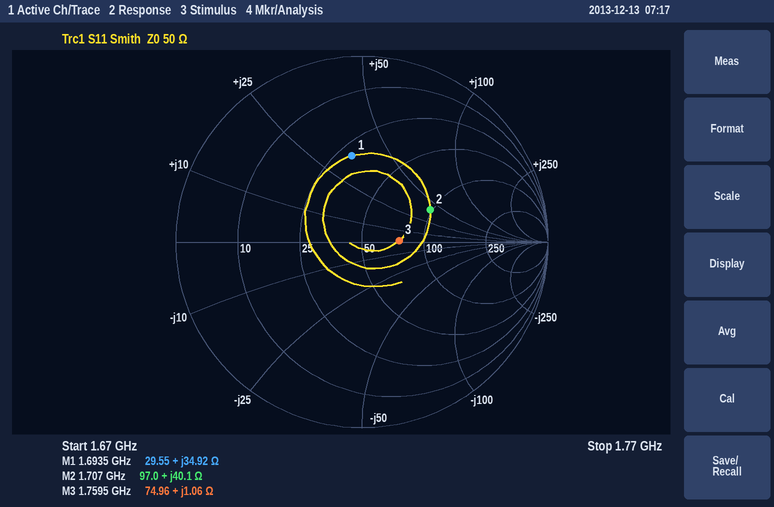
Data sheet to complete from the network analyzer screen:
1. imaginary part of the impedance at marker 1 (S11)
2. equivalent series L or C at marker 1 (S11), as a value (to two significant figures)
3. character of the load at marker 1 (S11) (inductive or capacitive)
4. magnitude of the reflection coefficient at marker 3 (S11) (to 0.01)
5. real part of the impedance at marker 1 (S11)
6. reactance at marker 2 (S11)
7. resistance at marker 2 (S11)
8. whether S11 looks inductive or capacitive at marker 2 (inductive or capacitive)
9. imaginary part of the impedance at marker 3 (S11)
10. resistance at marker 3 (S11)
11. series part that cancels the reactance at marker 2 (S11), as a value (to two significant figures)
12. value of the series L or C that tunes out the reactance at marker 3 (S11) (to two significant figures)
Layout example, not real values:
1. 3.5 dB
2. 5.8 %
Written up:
1. +34.92 Ω
2. 3.3 nH
3. inductive
4. 0.20
5. 29.55 Ω
6. +40.1 Ω
7. 97.0 Ω
8. inductive
9. +1.06 Ω
10. 74.96 Ω
11. 2.3 pF
12. 85 pF
